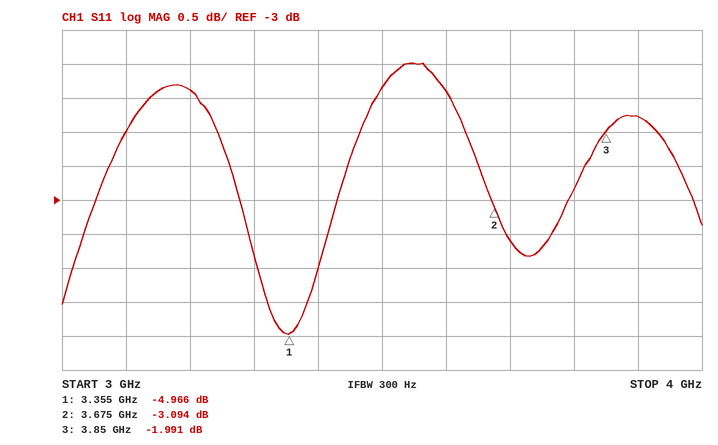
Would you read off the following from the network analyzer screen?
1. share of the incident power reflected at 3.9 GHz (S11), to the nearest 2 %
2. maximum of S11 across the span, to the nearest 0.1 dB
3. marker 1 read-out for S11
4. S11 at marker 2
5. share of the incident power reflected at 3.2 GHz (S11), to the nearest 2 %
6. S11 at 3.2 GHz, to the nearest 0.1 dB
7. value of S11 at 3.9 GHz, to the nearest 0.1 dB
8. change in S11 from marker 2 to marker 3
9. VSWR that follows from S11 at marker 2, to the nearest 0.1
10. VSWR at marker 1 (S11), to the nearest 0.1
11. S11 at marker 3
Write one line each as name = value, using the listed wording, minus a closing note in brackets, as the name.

share of the incident power reflected at 3.9 GHz (S11), to the nearest 2 % = 66 %
maximum of S11 across the span, to the nearest 0.1 dB = -1.0 dB
marker 1 read-out for S11 = -4.966 dB
S11 at marker 2 = -3.094 dB
share of the incident power reflected at 3.2 GHz (S11), to the nearest 2 % = 72 %
S11 at 3.2 GHz, to the nearest 0.1 dB = -1.4 dB
value of S11 at 3.9 GHz, to the nearest 0.1 dB = -1.8 dB
change in S11 from marker 2 to marker 3 = 1.103 dB
VSWR that follows from S11 at marker 2, to the nearest 0.1 = 5.7
VSWR at marker 1 (S11), to the nearest 0.1 = 3.6
S11 at marker 3 = -1.991 dB
